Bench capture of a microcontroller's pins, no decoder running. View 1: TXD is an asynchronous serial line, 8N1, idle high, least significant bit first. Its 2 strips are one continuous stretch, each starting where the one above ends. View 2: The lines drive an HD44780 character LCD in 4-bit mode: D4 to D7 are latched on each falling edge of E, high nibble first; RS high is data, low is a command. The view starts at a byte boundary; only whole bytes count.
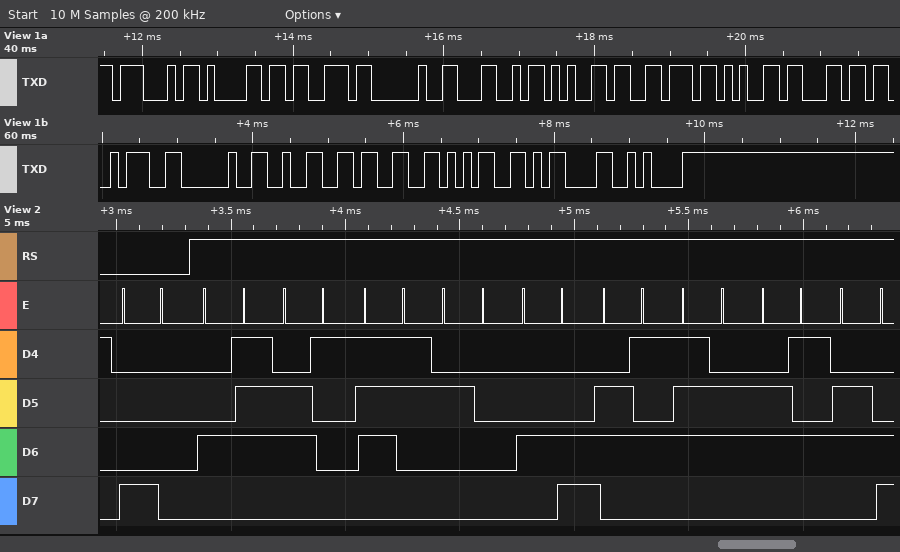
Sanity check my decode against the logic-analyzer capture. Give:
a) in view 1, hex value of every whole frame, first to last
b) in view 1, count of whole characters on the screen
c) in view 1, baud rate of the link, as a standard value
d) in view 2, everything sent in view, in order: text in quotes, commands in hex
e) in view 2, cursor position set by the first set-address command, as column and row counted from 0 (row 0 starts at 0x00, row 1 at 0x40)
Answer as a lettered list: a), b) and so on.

a) 47 61 73 20 4C 65 76 65 6C 3A 20 32 33 35 0D 0A
b) 16
c) 9600 baud
d) 0x80 "Gas Level"
e) column 0, row 0
